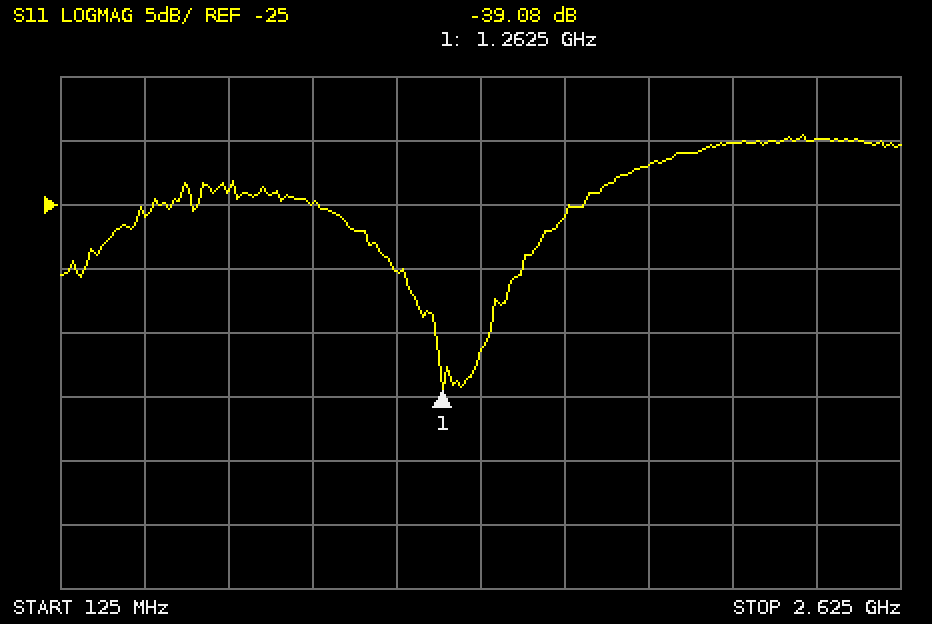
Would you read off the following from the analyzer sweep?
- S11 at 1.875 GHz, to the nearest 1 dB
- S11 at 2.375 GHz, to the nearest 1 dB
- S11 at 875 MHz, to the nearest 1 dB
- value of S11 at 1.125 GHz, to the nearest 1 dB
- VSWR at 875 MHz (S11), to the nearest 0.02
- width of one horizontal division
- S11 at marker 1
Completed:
-22 dB
-20 dB
-25 dB
-30 dB
1.12
250 MHz
-39.08 dB
